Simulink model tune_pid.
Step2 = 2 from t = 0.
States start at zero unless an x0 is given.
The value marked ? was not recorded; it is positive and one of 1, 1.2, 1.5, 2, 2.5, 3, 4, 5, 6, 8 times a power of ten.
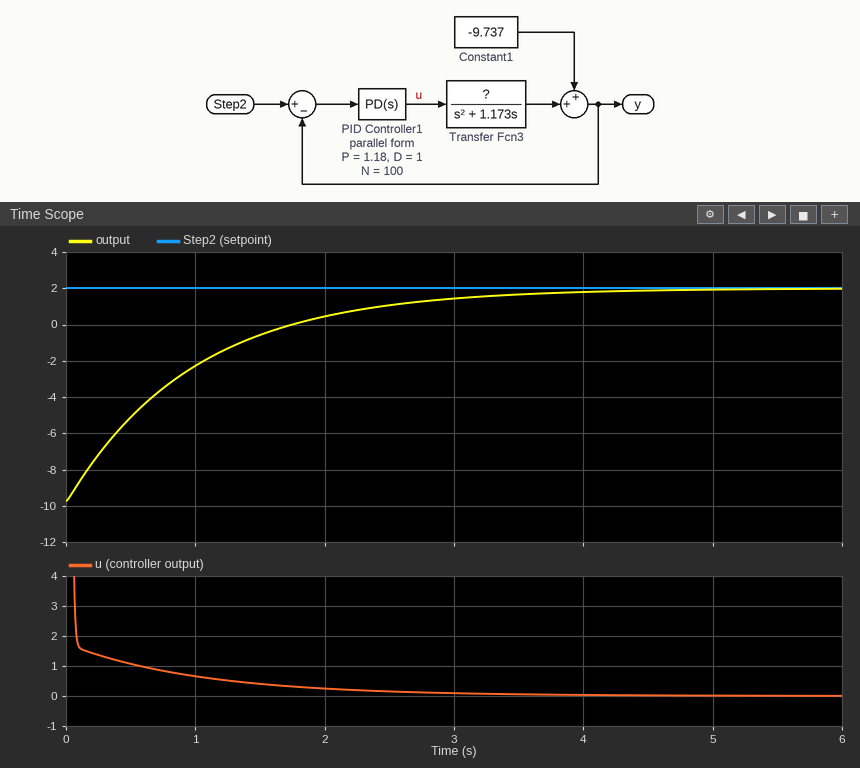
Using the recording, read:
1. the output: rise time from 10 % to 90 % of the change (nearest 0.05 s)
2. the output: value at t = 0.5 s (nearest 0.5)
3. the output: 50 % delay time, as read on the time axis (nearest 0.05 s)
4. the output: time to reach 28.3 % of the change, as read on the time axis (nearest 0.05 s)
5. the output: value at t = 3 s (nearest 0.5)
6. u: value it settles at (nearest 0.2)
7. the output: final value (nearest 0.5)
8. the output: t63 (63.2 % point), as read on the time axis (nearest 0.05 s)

2.15 s
-5.0
0.70 s
0.35 s
1.5
0.0
2.0
1.00 s
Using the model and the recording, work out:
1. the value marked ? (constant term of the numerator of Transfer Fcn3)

1
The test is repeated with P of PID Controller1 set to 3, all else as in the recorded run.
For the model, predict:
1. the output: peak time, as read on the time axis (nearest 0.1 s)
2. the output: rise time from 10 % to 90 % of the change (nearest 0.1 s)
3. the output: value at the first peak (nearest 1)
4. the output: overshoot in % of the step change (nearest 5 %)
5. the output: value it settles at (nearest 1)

1.9 s
0.9 s
3
10 %
2
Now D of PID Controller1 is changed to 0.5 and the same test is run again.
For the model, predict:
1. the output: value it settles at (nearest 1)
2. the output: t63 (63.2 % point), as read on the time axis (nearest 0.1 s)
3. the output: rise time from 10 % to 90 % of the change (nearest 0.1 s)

2
1.2 s
1.9 s
